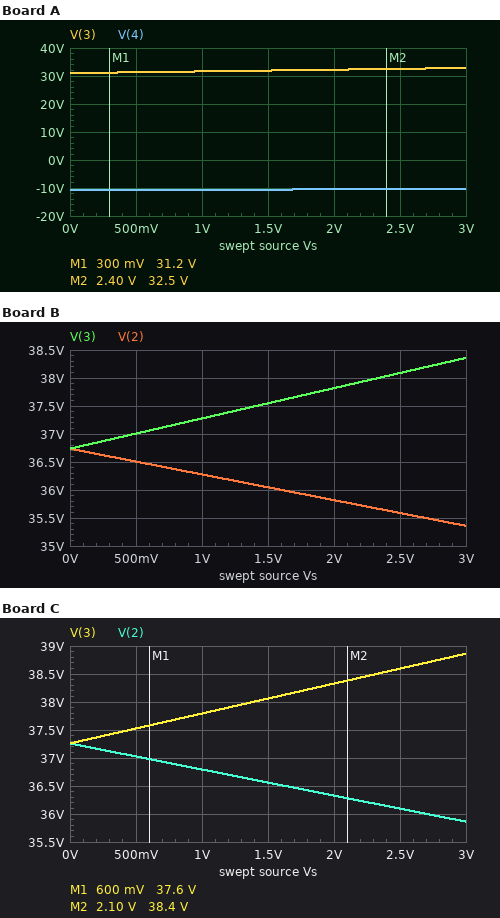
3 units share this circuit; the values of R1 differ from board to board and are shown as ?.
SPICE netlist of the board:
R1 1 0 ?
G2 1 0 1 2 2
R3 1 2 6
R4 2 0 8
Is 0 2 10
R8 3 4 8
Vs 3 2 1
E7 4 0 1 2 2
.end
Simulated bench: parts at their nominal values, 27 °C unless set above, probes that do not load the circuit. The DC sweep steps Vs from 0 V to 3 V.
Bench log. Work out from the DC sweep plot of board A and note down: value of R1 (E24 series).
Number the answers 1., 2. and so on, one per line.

1. 2.2 Ω
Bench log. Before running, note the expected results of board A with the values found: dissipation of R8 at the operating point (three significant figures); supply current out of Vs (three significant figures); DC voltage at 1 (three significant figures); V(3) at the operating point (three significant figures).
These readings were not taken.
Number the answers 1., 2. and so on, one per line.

1. 223 W
2. 5.28 A
3. 25.3 V
4. 31.6 V
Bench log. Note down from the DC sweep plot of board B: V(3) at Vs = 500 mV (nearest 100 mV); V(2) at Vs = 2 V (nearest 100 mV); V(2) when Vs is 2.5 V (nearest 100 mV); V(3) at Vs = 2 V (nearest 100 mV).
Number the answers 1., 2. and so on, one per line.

1. 37.0 V
2. 35.8 V
3. 35.6 V
4. 37.8 V
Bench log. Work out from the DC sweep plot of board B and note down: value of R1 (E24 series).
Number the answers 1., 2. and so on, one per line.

1. 8.2 Ω
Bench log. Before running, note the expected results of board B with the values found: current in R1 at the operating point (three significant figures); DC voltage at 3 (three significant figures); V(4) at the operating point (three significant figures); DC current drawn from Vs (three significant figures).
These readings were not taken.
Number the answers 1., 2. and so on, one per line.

1. 4.19 A
2. 37.3 V
3. -3.87 V
4. 5.14 A
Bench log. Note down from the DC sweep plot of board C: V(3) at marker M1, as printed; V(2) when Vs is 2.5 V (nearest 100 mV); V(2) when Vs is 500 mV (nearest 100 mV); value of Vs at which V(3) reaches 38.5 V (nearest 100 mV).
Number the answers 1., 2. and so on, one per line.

1. 37.6 V
2. 36.1 V
3. 37.0 V
4. 2.3 V
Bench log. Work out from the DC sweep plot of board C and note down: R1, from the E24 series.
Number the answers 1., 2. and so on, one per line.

1. 10 Ω
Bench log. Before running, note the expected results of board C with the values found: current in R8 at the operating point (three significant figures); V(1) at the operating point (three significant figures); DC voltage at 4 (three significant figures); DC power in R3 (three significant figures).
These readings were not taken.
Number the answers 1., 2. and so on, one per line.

1. 5.13 A
2. 35.2 V
3. -3.25 V
4. 439 mW
